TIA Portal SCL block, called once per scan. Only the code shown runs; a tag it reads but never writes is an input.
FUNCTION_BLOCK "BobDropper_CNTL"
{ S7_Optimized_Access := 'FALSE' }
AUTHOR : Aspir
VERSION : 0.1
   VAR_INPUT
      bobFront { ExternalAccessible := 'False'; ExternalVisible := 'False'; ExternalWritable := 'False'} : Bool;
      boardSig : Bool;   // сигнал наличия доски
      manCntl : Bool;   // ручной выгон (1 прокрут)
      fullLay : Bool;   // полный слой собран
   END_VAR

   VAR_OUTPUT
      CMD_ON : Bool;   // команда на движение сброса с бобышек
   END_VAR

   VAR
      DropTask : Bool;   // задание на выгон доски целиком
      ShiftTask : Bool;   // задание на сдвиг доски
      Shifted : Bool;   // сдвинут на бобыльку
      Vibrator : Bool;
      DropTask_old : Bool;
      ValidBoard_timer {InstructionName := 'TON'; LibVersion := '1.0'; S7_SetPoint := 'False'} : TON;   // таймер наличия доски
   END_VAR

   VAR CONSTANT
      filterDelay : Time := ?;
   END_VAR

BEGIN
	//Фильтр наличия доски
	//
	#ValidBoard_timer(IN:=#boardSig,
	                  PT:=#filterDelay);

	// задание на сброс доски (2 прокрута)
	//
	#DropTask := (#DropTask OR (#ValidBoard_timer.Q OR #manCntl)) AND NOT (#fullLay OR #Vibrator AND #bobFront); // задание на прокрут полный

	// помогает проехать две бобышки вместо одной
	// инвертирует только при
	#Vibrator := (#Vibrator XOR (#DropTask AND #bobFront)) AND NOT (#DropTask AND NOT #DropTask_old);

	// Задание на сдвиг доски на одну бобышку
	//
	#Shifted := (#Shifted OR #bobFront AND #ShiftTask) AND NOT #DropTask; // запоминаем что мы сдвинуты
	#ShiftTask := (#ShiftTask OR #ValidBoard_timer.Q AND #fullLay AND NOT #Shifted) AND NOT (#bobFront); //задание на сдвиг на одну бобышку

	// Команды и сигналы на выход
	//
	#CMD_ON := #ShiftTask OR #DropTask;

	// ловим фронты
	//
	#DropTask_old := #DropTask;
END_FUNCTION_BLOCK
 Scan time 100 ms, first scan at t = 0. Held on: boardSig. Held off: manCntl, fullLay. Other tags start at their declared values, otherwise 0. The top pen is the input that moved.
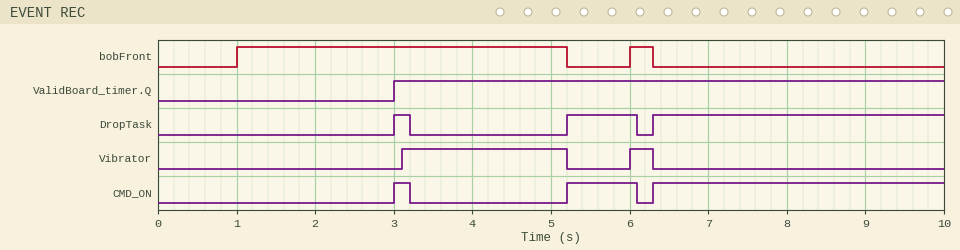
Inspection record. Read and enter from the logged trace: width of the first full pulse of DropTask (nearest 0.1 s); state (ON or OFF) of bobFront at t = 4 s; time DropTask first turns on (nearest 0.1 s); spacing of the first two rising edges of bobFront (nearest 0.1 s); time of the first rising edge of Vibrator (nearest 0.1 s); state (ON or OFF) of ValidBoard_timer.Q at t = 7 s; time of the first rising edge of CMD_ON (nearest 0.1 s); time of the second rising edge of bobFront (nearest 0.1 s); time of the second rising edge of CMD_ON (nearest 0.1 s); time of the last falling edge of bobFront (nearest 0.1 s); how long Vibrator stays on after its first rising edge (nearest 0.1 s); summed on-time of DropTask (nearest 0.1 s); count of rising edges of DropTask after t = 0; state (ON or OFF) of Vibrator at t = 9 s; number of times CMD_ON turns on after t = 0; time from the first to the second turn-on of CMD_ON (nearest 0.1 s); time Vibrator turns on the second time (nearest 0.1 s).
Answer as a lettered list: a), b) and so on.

a) 0.2 s
b) ON
c) 3.0 s
d) 5.0 s
e) 3.1 s
f) ON
g) 3.0 s
h) 6.0 s
i) 5.2 s
j) 6.3 s
k) 2.1 s
l) 4.8 s
m) 3
n) OFF
o) 3
p) 2.2 s
q) 6.0 s
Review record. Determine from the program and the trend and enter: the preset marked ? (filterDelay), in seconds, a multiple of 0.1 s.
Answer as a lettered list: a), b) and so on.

a) 3.0 s
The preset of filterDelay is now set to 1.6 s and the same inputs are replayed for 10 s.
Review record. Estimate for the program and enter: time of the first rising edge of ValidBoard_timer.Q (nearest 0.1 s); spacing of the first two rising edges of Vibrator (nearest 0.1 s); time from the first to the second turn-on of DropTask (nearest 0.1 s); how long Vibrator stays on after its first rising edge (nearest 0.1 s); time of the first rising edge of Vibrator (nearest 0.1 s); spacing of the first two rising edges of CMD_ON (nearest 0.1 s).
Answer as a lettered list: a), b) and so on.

a) 1.6 s
b) 4.3 s
c) 3.6 s
d) 3.5 s
e) 1.7 s
f) 3.6 s
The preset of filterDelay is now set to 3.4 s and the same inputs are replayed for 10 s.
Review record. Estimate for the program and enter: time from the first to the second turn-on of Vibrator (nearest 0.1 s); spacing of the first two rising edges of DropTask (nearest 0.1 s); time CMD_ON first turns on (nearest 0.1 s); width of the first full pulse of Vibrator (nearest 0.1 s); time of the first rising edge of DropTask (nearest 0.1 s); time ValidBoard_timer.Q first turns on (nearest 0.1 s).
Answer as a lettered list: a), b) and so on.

a) 2.5 s
b) 1.8 s
c) 3.4 s
d) 1.7 s
e) 3.4 s
f) 3.4 s
